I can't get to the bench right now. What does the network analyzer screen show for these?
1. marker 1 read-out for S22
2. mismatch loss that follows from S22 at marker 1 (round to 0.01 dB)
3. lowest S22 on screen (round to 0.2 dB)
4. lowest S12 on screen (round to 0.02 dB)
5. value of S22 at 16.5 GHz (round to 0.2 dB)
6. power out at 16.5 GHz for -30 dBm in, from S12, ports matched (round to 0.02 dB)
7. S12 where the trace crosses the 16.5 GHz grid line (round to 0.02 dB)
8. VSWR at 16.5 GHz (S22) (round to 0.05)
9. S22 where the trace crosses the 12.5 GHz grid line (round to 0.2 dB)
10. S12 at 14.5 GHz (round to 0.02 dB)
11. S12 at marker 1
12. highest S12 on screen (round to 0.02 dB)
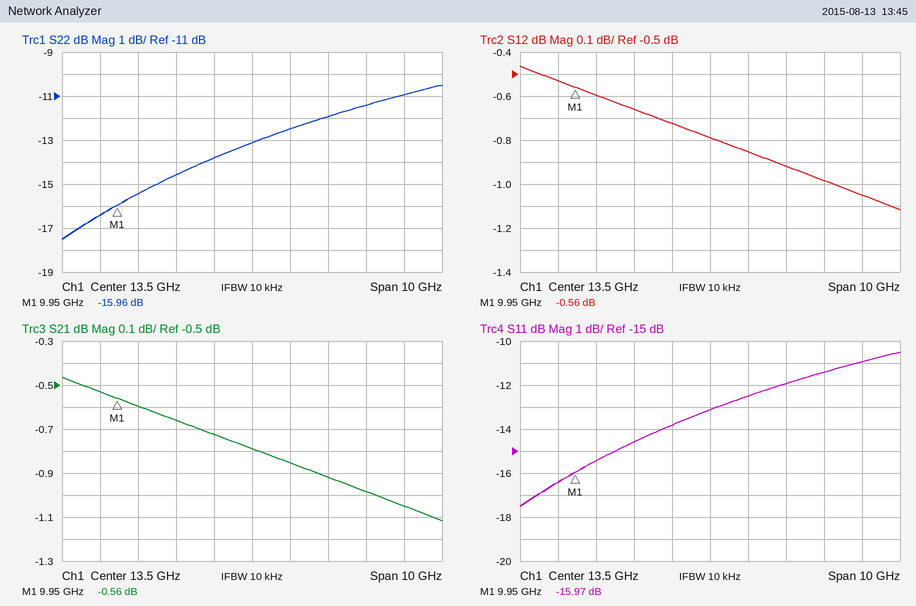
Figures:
-15.96 dB
0.11 dB
-17.6 dB
-1.12 dB
-11.4 dB
-30.98 dBm
-0.98 dB
1.75
-13.8 dB
-0.86 dB
-0.56 dB
-0.46 dB
